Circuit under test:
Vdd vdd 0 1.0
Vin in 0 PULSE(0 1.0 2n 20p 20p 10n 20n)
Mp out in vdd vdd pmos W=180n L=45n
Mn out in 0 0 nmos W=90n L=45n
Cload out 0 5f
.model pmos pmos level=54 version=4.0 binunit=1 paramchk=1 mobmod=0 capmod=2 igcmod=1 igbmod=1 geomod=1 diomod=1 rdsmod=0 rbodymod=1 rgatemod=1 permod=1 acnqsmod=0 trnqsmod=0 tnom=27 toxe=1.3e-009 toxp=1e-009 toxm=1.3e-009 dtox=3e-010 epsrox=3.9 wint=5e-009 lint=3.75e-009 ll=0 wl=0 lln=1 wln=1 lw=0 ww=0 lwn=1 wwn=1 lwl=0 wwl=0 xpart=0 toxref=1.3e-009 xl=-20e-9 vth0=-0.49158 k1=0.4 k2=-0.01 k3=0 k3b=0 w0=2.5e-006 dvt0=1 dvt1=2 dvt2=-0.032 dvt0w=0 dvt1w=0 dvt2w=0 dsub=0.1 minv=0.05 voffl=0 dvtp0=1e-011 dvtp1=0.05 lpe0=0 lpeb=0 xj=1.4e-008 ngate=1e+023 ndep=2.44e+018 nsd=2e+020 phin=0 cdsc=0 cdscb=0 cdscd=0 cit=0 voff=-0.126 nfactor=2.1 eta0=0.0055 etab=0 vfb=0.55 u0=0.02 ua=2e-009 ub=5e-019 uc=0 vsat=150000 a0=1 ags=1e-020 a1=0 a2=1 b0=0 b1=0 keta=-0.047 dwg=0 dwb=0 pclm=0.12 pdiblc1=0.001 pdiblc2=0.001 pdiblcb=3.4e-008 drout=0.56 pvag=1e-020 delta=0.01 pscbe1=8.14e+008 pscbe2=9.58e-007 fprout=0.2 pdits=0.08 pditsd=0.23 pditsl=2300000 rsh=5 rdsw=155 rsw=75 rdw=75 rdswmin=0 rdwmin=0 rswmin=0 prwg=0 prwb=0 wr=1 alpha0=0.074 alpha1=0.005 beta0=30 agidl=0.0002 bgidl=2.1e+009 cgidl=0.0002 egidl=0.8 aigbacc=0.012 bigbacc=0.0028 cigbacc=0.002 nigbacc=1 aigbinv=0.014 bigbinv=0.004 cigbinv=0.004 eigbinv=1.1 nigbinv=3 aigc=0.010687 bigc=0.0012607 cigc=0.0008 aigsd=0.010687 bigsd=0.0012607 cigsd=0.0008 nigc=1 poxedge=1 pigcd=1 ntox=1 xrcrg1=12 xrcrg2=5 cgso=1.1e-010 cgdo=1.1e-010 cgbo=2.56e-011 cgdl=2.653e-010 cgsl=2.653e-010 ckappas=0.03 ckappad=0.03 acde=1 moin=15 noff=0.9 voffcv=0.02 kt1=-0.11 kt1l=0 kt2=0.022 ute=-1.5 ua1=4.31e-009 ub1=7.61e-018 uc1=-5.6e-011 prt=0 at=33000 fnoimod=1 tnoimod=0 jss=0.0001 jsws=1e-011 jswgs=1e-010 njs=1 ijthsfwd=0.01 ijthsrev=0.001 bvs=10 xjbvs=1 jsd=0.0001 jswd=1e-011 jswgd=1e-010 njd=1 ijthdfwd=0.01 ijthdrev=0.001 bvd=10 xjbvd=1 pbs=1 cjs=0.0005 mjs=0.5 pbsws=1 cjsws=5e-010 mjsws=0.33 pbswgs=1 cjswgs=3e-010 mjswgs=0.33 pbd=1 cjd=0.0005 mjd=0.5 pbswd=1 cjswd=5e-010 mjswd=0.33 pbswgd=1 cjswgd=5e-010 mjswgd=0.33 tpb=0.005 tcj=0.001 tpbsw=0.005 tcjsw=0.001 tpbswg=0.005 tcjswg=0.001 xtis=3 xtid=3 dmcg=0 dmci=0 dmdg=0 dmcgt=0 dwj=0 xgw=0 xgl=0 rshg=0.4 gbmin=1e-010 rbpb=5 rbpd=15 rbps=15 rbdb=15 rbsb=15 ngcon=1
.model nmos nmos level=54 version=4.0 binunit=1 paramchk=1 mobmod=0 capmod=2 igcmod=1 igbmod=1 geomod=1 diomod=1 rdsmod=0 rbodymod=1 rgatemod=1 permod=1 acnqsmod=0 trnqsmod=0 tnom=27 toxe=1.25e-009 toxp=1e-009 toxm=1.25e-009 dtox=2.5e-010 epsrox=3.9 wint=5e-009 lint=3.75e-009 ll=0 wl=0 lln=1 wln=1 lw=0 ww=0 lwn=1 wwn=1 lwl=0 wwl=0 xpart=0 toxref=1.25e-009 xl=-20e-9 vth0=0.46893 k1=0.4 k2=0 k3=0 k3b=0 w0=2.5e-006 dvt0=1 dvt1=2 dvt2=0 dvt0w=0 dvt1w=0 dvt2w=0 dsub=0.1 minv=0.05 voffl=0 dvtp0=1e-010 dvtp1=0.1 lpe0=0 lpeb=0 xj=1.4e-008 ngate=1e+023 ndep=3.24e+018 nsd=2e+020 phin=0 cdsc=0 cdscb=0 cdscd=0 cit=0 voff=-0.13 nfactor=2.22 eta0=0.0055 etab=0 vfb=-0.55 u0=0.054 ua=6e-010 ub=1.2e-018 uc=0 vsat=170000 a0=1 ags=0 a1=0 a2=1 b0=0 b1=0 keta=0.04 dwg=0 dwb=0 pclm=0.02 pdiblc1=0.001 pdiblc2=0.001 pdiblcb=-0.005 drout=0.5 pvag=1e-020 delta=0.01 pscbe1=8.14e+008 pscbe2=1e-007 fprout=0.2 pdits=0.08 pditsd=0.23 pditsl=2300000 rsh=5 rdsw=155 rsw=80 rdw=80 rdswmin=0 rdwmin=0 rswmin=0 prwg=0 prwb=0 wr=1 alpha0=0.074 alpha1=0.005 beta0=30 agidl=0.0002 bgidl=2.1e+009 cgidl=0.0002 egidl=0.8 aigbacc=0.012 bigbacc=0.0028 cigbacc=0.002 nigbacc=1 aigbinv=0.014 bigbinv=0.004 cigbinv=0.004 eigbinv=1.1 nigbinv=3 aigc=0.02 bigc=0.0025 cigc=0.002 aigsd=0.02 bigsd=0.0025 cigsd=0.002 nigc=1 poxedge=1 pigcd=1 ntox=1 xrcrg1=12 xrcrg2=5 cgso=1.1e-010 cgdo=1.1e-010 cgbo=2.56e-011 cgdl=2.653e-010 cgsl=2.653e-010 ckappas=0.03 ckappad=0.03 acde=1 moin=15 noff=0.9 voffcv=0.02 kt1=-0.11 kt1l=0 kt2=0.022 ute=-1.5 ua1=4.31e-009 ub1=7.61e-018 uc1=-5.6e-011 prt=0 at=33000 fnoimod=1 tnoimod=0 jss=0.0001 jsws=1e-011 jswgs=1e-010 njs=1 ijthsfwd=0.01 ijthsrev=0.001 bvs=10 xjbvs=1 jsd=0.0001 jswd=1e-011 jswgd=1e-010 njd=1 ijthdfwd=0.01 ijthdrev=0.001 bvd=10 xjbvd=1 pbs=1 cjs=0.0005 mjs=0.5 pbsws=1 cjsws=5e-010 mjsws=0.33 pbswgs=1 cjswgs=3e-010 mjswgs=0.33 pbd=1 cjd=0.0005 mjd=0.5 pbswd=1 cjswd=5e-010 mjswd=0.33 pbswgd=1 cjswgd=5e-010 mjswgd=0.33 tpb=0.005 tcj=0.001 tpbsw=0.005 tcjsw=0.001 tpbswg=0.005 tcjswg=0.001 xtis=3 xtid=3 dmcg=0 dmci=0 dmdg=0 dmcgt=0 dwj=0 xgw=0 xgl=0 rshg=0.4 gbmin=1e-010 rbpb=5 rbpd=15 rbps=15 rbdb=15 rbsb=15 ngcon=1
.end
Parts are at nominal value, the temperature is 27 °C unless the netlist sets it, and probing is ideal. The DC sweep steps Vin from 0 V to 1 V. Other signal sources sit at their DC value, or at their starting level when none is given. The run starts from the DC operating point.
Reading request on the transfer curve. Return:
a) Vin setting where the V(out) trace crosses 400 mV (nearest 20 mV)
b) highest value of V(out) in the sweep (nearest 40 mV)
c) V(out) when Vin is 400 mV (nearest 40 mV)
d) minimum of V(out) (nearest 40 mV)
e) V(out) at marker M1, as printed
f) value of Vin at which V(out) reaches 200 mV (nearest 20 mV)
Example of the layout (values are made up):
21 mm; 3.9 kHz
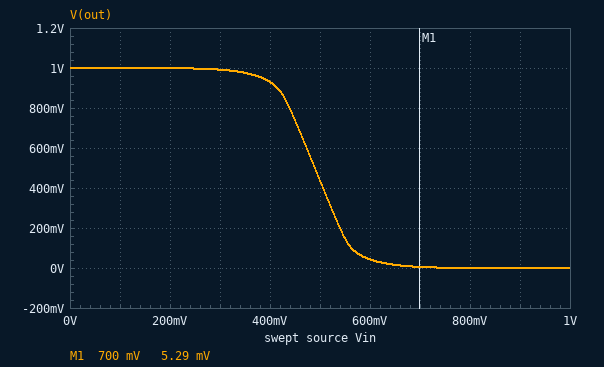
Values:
500 mV; 1.00 V; 920 mV; 0 V; 5.29 mV; 540 mV
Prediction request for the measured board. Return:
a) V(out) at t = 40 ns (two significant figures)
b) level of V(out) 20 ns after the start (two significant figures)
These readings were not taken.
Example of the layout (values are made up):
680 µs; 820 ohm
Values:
1.0 V; 1.0 V
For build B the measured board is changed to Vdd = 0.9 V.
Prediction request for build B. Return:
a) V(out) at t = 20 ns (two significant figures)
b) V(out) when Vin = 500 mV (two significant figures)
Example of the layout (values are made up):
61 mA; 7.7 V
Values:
900 mV; 77 mV
